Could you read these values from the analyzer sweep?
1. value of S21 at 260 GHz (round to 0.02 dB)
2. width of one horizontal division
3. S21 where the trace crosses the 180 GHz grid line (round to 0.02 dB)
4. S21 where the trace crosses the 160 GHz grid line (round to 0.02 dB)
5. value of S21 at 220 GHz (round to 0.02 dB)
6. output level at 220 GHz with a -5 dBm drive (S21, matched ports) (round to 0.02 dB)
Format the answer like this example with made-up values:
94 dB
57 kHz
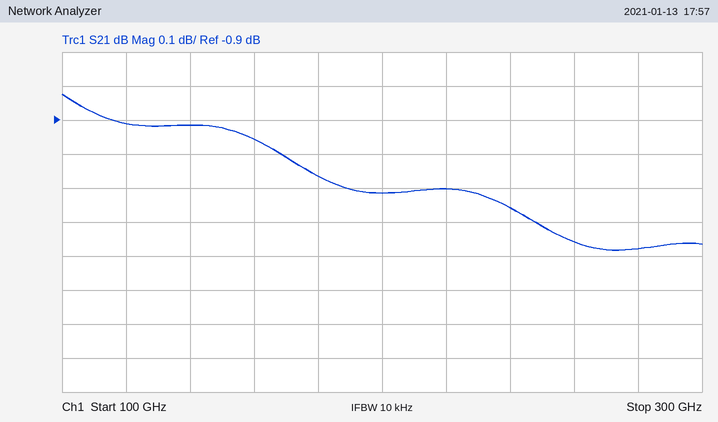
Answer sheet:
-1.26 dB
20 GHz
-1.06 dB
-0.96 dB
-1.10 dB
-6.10 dBm
